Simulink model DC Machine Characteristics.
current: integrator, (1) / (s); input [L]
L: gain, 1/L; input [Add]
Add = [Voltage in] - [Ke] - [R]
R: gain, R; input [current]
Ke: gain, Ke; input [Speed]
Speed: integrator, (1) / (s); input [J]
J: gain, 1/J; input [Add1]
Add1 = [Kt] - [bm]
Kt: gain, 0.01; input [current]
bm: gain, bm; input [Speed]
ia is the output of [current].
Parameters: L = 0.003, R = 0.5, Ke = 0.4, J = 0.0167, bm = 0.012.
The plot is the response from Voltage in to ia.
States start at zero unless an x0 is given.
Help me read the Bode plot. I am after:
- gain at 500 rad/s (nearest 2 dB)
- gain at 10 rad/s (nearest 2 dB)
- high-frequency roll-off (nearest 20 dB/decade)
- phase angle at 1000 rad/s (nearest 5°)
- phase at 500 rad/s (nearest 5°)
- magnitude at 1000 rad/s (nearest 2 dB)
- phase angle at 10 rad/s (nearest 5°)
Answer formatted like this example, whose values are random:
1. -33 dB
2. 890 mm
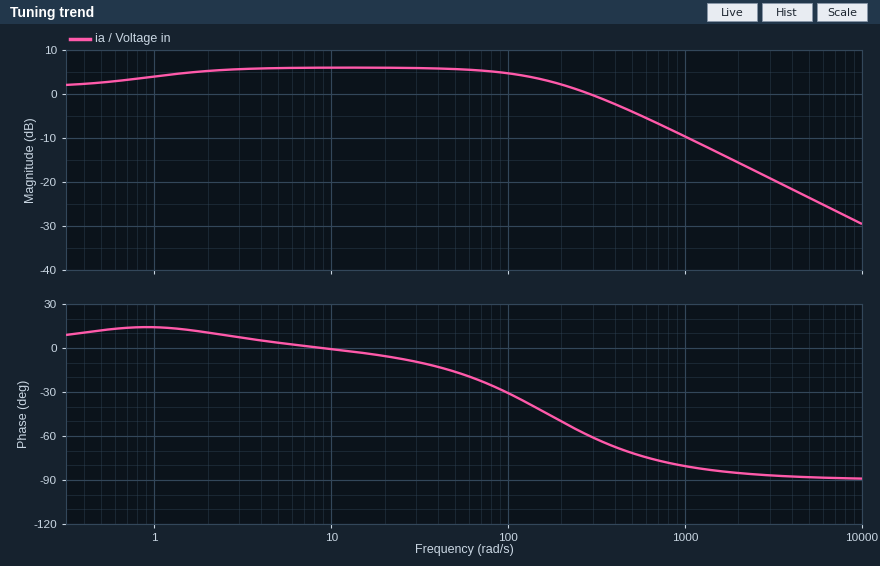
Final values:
1. -4 dB
2. 6 dB
3. -20 dB/decade
4. -80°
5. -70°
6. -10 dB
7. 0°
